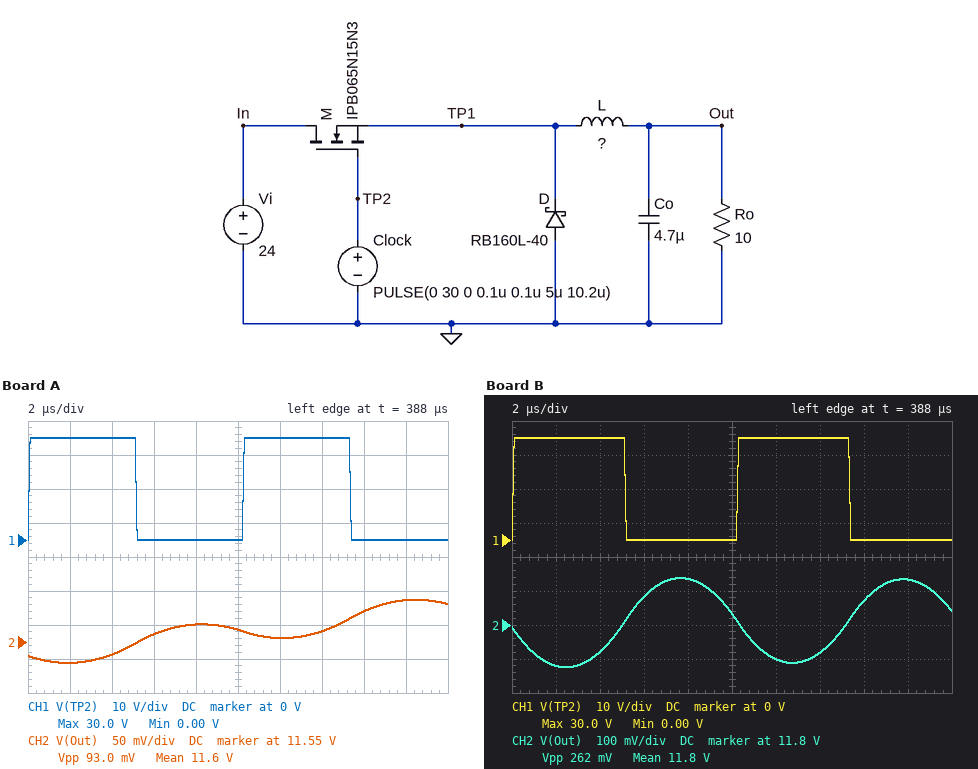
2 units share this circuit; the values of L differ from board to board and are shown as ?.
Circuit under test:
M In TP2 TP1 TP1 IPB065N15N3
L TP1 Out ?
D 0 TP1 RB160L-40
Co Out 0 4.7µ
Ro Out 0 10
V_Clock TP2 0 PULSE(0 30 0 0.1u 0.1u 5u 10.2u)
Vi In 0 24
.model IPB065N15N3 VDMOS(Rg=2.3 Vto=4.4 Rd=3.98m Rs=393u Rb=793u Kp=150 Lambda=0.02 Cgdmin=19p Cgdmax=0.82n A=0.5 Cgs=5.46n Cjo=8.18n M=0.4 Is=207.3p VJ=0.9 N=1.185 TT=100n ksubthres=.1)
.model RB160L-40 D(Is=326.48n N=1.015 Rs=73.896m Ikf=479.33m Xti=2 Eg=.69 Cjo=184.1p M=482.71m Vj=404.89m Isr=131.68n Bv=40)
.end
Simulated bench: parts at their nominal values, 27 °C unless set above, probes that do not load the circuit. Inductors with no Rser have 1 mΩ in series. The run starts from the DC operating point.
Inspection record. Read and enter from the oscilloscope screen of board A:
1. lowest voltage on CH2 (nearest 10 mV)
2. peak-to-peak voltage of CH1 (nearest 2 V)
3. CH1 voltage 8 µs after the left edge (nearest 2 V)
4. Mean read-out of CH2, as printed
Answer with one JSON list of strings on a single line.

["11.52 V", "30 V", "0 V", "11.6 V"]
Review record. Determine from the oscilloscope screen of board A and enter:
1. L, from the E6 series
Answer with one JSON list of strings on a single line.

["470 µH"]
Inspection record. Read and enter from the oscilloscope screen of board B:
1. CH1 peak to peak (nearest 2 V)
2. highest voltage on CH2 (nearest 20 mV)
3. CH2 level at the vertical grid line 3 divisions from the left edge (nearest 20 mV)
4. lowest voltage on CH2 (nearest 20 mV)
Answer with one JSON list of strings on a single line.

["30 V", "11.94 V", "11.88 V", "11.68 V"]
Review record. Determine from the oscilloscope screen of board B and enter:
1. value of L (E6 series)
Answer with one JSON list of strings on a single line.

["68 µH"]
